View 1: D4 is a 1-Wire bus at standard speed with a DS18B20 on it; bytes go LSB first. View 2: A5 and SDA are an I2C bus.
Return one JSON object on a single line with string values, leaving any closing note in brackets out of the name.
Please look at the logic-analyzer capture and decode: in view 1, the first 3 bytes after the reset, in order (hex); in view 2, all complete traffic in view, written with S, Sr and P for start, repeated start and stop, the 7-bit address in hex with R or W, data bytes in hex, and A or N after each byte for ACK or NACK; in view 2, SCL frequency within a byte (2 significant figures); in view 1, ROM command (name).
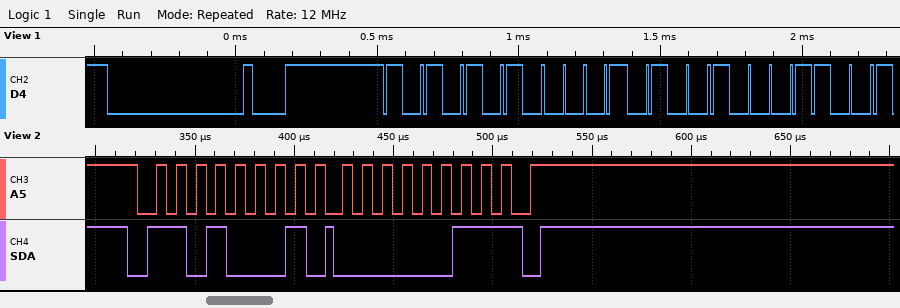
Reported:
{"in view 1, the first 3 bytes after the reset, in order": "55 28 31", "in view 2, all complete traffic in view, written with S, Sr and P for start, repeated start and stop, the 7-bit address in hex with R or W, data bytes in hex, and A or N after each byte for ACK or NACK": "S 68R A 03 N P", "in view 2, SCL frequency within a byte": "100 kHz", "in view 1, ROM command": "Match ROM"}
